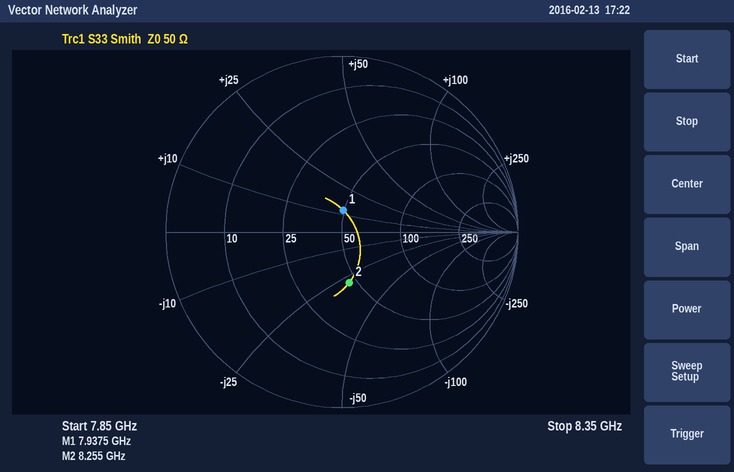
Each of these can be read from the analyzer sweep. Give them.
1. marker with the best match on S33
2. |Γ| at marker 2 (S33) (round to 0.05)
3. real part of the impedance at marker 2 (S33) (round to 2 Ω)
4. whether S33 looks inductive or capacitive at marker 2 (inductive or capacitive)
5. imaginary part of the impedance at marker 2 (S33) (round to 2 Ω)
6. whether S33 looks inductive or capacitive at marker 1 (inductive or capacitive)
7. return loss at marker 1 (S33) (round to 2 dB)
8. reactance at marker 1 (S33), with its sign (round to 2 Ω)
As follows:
marker 1
0.30
46 Ω
capacitive
-28 Ω
inductive
18 dB
+12 Ω
